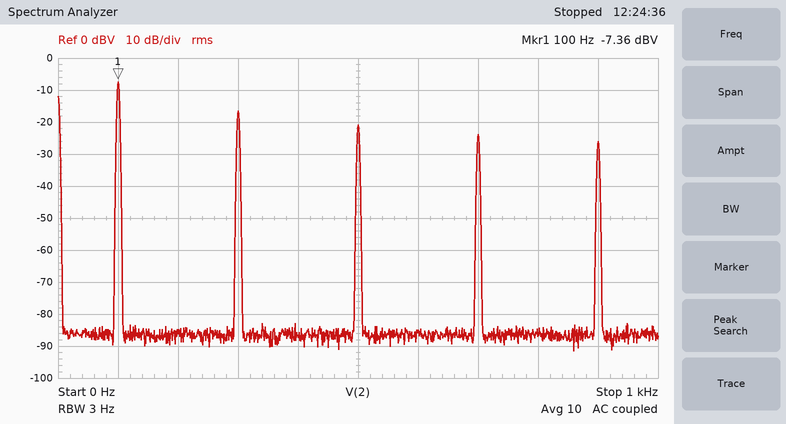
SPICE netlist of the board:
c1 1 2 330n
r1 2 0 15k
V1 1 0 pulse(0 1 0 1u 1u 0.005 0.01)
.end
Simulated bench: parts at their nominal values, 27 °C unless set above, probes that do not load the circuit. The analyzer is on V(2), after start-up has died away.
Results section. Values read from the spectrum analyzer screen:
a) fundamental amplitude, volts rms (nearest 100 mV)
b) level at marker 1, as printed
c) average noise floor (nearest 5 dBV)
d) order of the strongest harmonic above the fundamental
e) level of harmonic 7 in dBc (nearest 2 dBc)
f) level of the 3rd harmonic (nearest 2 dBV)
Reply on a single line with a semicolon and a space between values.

400 mV; -7.36 dBV; -85 dBV; 3; -16 dBc; -16 dBV
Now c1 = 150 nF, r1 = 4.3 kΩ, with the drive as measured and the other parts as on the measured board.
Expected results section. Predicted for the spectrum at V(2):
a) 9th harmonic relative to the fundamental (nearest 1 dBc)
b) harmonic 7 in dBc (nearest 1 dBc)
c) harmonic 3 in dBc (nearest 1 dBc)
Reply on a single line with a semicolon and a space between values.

-11 dBc; -9 dBc; -3 dBc
